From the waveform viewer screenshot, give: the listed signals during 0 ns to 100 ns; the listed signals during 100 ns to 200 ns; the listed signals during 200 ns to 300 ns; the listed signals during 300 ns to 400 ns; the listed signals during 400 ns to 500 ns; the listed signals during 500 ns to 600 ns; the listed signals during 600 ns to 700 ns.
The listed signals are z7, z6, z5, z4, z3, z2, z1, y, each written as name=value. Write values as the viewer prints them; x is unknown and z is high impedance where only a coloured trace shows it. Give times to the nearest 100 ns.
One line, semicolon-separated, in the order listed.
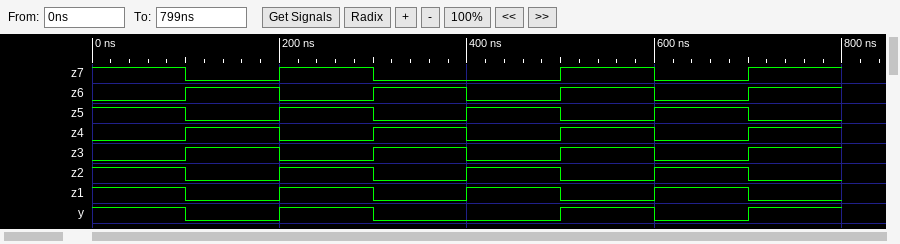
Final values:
z7=1, z6=0, z5=1, z4=0, z3=0, z2=1, z1=1, y=1; z7=0, z6=1, z5=0, z4=1, z3=1, z2=0, z1=0, y=0; z7=1, z6=0, z5=1, z4=0, z3=0, z2=1, z1=1, y=1; z7=0, z6=1, z5=0, z4=1, z3=1, z2=0, z1=0, y=0; z7=0, z6=0, z5=1, z4=0, z3=0, z2=1, z1=1, y=0; z7=1, z6=1, z5=0, z4=1, z3=1, z2=0, z1=0, y=1; z7=0, z6=0, z5=1, z4=0, z3=0, z2=1, z1=1, y=0
